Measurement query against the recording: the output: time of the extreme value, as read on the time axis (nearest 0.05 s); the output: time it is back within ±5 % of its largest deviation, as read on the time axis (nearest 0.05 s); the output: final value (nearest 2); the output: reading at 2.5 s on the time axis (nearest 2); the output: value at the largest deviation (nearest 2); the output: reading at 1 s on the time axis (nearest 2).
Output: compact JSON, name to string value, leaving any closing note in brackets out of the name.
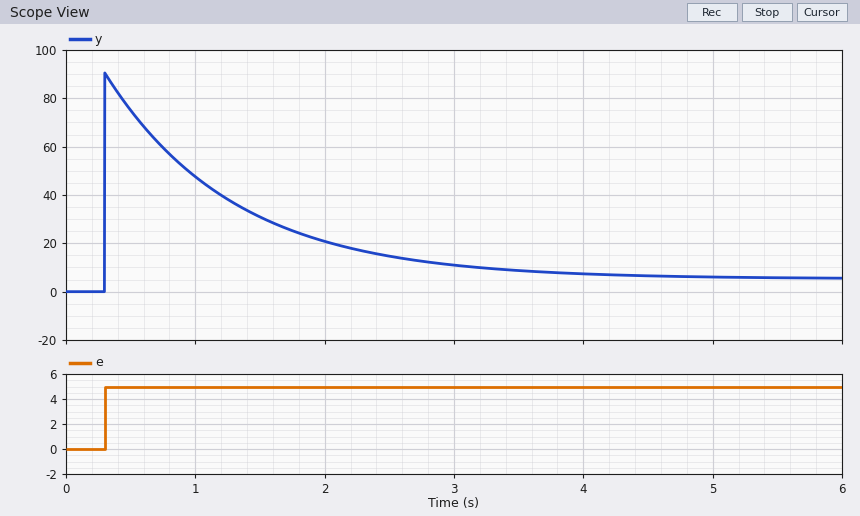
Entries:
{"the output: time of the extreme value, as read on the time axis": "0.30 s", "the output: time it is back within ±5 % of its largest deviation, as read on the time axis": "3.15 s", "the output: final value": "6", "the output: reading at 2.5 s on the time axis": "14", "the output: value at the largest deviation": "90", "the output: reading at 1 s on the time axis": "48"}
